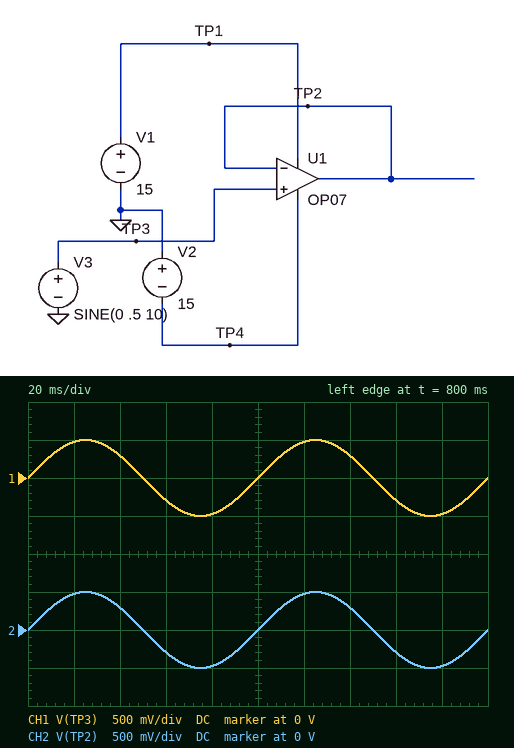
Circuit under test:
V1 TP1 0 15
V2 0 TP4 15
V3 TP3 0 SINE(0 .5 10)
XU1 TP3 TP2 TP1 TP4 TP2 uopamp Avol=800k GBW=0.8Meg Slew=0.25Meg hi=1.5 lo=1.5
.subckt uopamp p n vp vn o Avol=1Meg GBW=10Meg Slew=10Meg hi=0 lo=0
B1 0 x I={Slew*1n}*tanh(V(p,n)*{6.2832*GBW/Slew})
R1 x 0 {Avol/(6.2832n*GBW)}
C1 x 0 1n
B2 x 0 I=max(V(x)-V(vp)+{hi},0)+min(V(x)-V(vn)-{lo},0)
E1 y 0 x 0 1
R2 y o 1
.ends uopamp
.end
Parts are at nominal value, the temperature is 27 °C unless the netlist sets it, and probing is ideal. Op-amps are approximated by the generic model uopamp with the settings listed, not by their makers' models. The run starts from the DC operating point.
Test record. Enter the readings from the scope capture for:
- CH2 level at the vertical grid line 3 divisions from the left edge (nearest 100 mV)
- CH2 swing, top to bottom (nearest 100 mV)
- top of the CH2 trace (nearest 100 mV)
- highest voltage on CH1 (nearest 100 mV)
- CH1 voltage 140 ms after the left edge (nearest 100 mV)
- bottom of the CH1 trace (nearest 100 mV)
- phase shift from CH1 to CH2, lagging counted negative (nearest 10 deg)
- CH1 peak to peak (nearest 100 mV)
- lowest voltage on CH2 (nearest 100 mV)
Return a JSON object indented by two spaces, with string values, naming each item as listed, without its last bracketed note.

{
  "CH2 level at the vertical grid line 3 divisions from the left edge": "-300 mV",
  "CH2 swing, top to bottom": "1.0 V",
  "top of the CH2 trace": "500 mV",
  "highest voltage on CH1": "500 mV",
  "CH1 voltage 140 ms after the left edge": "300 mV",
  "bottom of the CH1 trace": "-500 mV",
  "phase shift from CH1 to CH2, lagging counted negative": "0 deg",
  "CH1 peak to peak": "1.0 V",
  "lowest voltage on CH2": "-500 mV"
}
